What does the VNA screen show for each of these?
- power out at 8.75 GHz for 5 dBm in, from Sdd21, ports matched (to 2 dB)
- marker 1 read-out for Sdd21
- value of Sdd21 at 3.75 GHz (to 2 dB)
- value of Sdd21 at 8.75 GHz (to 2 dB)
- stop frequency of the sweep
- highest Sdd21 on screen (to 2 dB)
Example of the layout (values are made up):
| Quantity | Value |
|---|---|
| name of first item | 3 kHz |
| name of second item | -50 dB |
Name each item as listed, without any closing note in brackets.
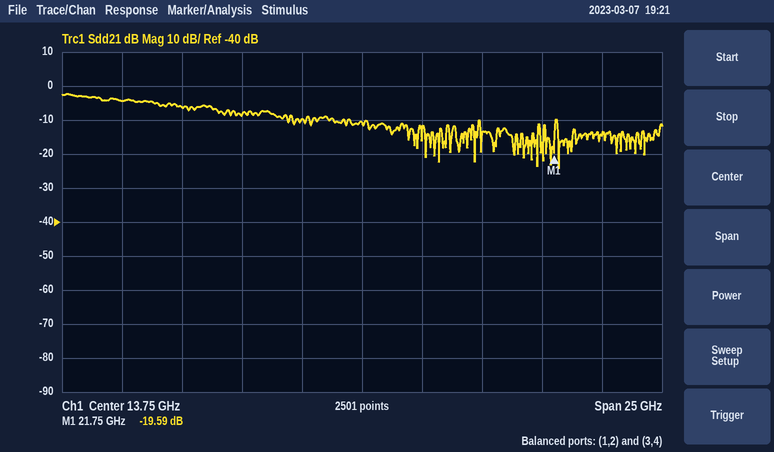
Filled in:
| Quantity | Value |
|---|---|
| power out at 8.75 GHz for 5 dBm in, from Sdd21, ports matched | -4 dBm |
| marker 1 read-out for Sdd21 | -19.59 dB |
| value of Sdd21 at 3.75 GHz | -4 dB |
| value of Sdd21 at 8.75 GHz | -8 dB |
| stop frequency of the sweep | 26.25 GHz |
| highest Sdd21 on screen | -2 dB |
